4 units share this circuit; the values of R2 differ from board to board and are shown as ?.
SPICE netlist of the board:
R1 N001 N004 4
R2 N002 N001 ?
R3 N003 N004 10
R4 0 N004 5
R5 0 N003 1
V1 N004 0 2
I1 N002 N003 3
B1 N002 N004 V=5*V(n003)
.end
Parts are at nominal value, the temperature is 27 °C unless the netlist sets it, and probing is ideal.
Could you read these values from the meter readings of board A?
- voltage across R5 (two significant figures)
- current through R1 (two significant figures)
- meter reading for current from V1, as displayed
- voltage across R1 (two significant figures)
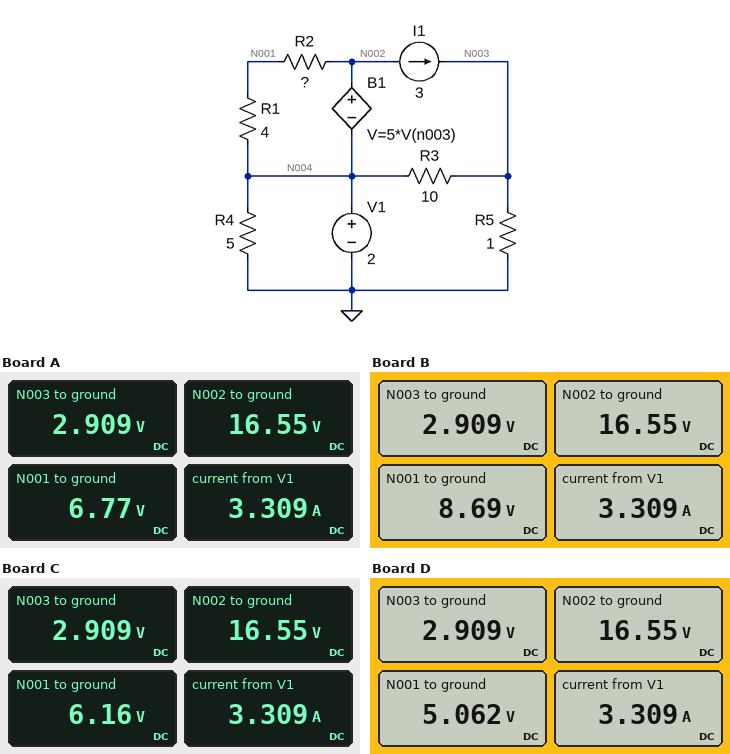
2.9 V
1.2 A
3.309 A
4.8 V
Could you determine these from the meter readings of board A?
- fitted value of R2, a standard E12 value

8.2 Ω
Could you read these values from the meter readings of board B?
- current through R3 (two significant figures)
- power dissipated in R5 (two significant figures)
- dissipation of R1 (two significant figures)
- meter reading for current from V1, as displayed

91 mA
8.5 W
11 W
3.309 A
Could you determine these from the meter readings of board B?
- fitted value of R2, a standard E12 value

4.7 Ω
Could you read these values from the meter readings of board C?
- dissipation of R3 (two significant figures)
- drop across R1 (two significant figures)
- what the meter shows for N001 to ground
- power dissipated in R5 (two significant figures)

83 mW
4.2 V
6.16 V
8.5 W
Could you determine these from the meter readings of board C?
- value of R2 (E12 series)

10 Ω
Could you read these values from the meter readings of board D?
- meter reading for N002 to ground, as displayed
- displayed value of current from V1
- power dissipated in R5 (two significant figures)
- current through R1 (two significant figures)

16.55 V
3.309 A
8.5 W
770 mA
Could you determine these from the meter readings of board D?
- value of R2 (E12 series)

15 Ω
